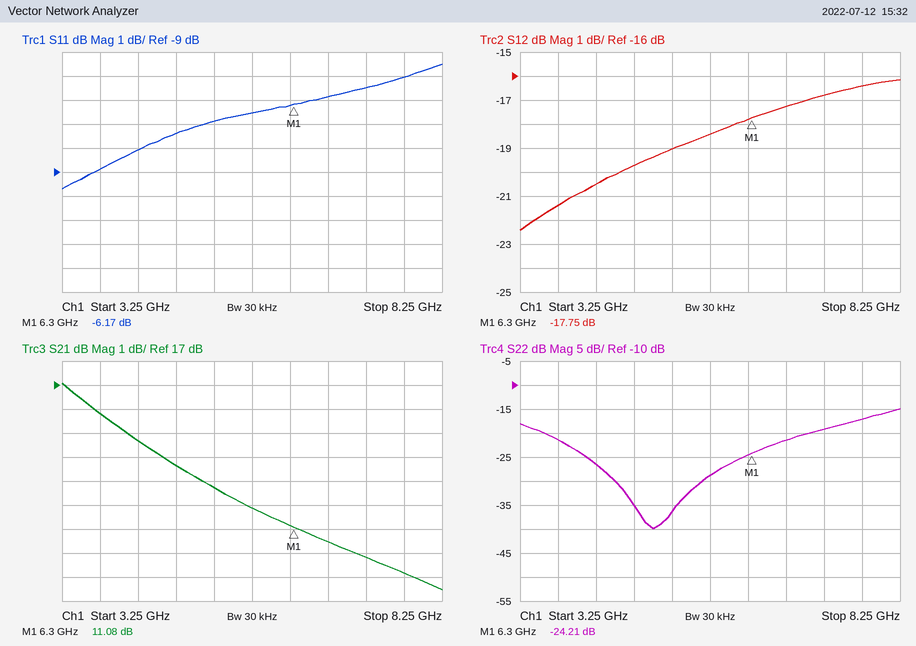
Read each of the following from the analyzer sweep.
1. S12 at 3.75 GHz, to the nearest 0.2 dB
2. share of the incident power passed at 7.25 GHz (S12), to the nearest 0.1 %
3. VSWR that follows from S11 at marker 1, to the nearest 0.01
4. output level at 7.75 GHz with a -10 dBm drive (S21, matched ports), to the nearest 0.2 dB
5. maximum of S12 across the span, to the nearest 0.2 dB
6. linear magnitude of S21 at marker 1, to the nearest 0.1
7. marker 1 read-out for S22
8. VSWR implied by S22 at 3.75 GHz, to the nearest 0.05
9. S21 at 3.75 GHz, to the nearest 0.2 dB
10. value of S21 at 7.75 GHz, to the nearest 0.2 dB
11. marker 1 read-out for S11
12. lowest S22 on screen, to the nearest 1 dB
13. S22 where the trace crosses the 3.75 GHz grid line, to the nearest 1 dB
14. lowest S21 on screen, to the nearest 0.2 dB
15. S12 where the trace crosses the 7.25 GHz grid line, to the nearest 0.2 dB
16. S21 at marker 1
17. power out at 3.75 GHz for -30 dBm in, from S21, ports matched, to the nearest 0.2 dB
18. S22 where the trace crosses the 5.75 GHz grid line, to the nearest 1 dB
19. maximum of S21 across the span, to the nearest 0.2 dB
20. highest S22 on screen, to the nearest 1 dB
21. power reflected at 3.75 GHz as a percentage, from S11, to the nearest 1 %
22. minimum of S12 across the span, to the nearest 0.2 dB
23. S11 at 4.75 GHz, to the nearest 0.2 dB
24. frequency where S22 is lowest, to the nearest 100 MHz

-21.4 dB
2.1 %
2.93
-0.8 dBm
-16.2 dB
3.6
-24.21 dB
1.20
15.8 dB
9.2 dB
-6.17 dB
-40 dB
-21 dB
8.4 dB
-16.8 dB
11.08 dB
-14.2 dBm
-29 dB
17.0 dB
-15 dB
13 %
-22.4 dB
-7.4 dB
5.0 GHz
